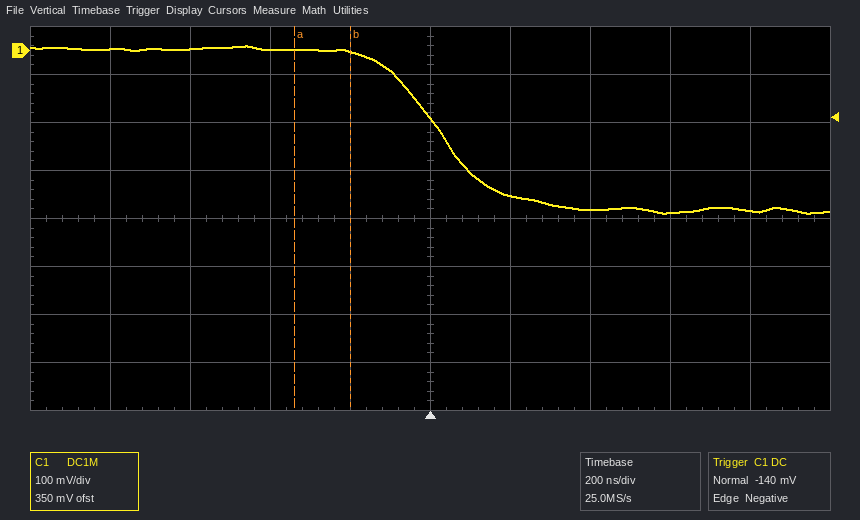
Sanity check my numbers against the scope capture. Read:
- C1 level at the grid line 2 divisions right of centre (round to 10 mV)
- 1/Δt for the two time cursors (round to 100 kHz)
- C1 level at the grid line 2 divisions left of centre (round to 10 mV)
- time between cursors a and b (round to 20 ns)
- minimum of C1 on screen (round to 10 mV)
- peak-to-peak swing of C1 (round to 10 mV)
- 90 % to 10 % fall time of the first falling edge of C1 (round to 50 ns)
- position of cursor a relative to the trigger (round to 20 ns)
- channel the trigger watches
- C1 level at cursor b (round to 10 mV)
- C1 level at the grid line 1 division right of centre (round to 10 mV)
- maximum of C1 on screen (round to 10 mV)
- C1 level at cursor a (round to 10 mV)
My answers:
-330 mV
7.1 MHz
0 mV
140 ns
-340 mV
350 mV
300 ns
-340 ns
C1
0 mV
-300 mV
10 mV
0 mV
